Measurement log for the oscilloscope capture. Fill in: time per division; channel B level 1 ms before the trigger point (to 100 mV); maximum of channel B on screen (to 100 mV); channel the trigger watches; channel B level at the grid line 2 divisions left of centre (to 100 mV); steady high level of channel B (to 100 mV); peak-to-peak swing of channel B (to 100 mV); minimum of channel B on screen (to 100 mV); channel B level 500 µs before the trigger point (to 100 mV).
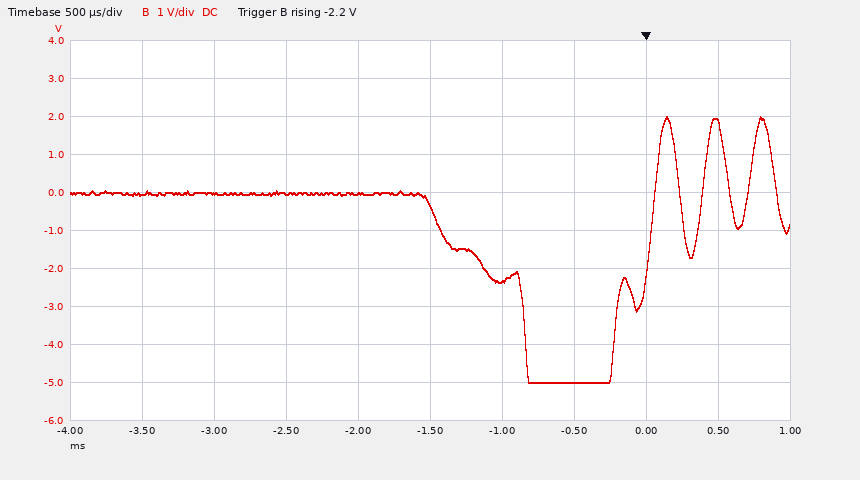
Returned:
500 µs
-2.3 V
2.0 V
channel B
0.0 V
0.0 V
7.0 V
-5.0 V
-5.0 V
